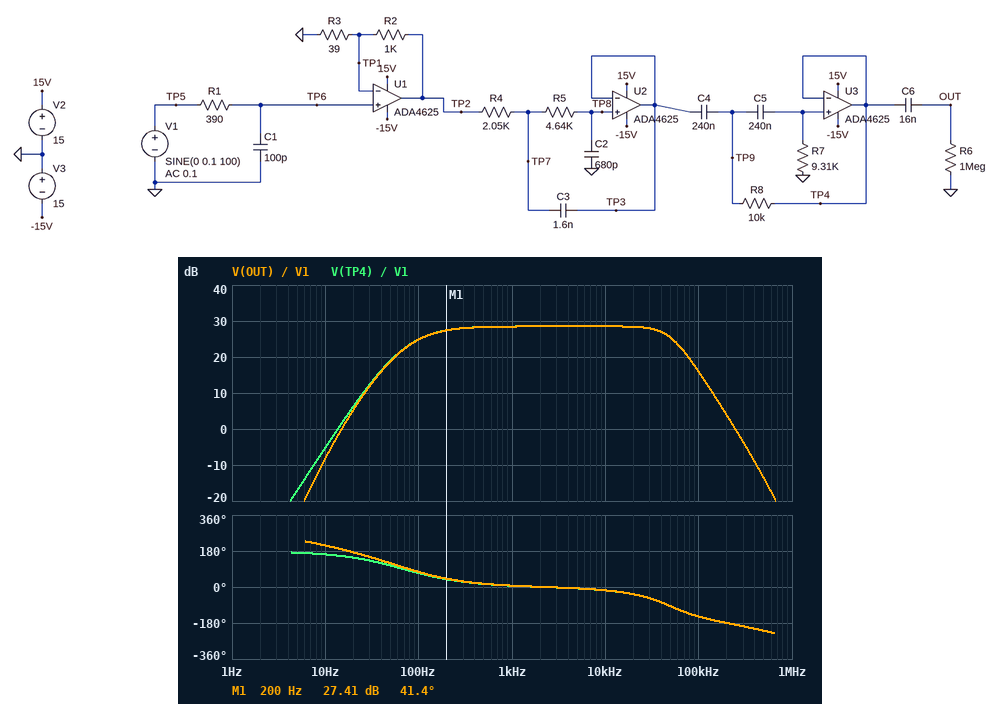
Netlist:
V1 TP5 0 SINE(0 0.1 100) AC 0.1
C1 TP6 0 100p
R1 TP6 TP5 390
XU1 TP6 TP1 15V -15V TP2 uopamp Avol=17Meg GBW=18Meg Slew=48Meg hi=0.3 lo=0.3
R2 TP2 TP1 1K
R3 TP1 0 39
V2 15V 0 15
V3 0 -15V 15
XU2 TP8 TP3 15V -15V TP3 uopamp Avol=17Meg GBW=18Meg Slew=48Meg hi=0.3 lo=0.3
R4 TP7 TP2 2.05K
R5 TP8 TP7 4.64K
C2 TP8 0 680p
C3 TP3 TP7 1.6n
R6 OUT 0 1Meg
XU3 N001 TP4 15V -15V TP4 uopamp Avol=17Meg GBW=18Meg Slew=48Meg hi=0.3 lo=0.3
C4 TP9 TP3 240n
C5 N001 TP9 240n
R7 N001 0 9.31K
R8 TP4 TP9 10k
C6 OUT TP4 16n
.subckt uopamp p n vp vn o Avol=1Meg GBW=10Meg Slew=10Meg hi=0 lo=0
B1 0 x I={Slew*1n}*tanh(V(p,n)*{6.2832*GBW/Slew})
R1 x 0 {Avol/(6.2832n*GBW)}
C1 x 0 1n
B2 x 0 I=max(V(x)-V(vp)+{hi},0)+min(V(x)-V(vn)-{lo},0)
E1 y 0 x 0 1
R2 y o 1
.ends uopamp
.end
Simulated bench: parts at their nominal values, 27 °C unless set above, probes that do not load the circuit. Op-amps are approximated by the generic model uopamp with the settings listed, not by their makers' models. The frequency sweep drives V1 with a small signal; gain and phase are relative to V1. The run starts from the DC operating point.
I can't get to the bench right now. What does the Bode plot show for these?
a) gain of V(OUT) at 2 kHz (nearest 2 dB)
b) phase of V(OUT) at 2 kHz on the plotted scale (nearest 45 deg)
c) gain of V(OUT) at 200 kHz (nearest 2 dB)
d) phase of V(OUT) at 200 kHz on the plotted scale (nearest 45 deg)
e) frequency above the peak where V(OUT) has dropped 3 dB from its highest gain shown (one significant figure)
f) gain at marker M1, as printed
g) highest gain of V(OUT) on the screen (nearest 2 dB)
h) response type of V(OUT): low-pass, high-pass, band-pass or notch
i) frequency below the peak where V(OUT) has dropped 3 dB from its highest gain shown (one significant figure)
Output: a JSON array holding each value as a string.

["28 dB", "0 deg", "4 dB", "-180 deg", "50 kHz", "27.41 dB", "28 dB", "band-pass", "100 Hz"]
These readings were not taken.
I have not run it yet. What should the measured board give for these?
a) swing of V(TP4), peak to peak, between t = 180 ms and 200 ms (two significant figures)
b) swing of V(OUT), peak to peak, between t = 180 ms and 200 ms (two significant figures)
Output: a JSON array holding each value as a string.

["3.5 V", "3.5 V"]
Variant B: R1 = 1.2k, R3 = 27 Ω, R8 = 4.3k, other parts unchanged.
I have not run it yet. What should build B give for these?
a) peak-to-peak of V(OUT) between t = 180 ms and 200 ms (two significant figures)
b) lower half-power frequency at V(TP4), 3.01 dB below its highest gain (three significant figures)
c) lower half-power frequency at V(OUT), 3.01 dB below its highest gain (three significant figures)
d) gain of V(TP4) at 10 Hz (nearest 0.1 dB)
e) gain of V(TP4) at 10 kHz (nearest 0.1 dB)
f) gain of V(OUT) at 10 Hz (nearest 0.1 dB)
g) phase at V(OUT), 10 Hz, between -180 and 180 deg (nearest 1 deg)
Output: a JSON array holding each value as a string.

["5.3 V", "101 Hz", "102 Hz", "-9.2 dB", "31.6 dB", "-12.2 dB", "-143 deg"]
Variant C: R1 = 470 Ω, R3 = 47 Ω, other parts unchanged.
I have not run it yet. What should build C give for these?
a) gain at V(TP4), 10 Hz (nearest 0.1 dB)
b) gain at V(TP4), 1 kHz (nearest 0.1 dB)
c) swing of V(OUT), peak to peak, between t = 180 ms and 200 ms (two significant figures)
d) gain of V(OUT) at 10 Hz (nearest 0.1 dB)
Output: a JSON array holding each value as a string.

["-6.7 dB", "26.9 dB", "2.9 V", "-9.7 dB"]
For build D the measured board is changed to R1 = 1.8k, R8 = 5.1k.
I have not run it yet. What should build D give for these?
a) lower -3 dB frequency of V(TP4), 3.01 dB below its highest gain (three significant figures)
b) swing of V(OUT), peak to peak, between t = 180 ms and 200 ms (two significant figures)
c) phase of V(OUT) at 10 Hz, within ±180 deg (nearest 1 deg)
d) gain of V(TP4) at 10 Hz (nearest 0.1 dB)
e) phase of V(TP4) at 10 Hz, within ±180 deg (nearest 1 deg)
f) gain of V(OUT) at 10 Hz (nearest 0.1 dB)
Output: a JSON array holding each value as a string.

["101 Hz", "3.7 V", "-144 deg", "-10.8 dB", "171 deg", "-13.8 dB"]
